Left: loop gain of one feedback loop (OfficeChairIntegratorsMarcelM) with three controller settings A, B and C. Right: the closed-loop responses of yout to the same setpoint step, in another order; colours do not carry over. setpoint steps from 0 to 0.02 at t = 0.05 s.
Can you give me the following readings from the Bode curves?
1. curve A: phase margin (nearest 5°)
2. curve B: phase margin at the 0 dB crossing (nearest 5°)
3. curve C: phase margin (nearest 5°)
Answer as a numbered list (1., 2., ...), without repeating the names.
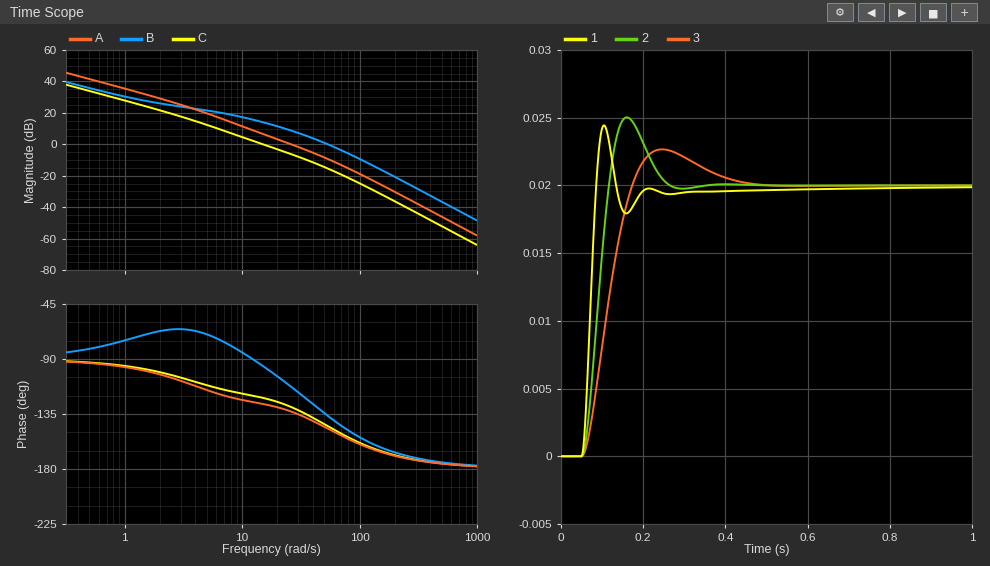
1. 45°
2. 45°
3. 60°
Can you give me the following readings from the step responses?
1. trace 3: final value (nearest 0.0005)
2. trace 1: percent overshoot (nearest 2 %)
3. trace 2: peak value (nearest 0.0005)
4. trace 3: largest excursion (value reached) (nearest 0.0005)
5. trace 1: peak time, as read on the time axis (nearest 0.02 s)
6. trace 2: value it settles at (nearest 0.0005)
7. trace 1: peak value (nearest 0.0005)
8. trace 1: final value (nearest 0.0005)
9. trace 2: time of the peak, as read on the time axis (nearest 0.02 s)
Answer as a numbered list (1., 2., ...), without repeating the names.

1. 0.0200
2. 22 %
3. 0.0250
4. 0.0225
5. 0.10 s
6. 0.0200
7. 0.0245
8. 0.0200
9. 0.16 s
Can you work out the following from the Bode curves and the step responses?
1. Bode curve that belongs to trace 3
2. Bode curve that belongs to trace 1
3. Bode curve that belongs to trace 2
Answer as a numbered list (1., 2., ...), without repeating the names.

1. C
2. B
3. A
